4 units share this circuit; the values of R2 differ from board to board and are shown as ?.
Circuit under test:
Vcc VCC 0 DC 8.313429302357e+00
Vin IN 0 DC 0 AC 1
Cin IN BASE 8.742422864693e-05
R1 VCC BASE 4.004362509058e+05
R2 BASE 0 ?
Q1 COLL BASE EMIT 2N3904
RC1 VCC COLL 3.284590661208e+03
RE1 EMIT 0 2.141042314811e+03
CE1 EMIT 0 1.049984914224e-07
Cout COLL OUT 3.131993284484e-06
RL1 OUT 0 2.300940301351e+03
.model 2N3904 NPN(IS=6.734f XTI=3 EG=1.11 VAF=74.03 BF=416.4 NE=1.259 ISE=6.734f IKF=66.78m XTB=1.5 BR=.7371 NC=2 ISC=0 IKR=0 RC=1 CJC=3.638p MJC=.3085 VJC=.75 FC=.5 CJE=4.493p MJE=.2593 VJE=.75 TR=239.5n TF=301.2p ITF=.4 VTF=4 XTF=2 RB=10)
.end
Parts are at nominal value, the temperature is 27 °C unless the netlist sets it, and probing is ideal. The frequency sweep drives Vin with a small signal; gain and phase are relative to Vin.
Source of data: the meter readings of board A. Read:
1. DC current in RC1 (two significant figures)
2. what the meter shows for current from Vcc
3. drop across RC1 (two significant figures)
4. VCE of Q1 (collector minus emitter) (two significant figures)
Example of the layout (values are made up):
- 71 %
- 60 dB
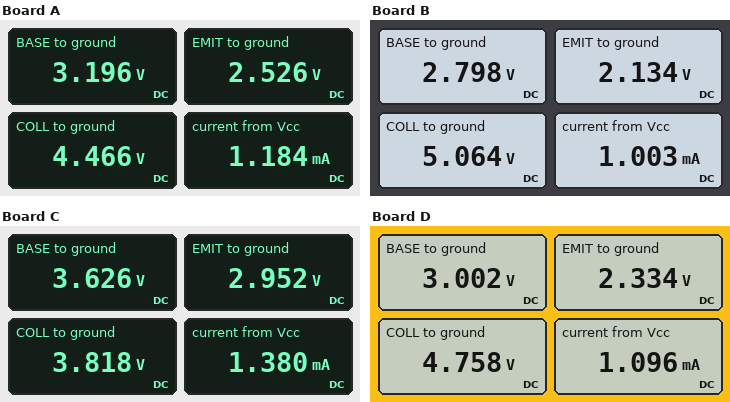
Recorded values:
- 1.2 mA
- 1.184 mA
- 3.8 V
- 1.9 V
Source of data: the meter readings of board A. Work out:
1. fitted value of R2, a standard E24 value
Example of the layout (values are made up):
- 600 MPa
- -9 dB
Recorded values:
- 750 kΩ
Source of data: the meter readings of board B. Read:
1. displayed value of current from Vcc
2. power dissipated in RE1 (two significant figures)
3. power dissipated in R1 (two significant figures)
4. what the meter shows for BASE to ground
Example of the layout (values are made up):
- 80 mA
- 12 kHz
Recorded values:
- 1.003 mA
- 2.1 mW
- 76 µW
- 2.798 V
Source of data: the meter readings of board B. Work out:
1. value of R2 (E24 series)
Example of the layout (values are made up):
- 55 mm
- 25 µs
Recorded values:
- 430 kΩ
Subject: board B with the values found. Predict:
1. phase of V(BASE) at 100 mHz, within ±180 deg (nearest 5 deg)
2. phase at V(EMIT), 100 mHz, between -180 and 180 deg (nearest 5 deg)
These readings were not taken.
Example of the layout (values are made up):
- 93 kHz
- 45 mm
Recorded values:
- 10 deg
- 10 deg
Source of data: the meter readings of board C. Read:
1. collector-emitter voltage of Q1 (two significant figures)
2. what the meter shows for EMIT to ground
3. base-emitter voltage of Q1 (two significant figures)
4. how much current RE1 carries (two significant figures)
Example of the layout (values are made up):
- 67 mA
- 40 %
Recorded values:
- 870 mV
- 2.952 V
- 670 mV
- 1.4 mA
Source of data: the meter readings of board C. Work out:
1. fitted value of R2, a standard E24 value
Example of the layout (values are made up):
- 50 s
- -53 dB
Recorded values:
- 2 MΩ
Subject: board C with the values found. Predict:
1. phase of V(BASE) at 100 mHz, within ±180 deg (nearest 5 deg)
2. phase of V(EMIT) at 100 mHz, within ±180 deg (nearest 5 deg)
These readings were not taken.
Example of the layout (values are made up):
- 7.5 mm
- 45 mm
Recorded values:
- 5 deg
- 5 deg
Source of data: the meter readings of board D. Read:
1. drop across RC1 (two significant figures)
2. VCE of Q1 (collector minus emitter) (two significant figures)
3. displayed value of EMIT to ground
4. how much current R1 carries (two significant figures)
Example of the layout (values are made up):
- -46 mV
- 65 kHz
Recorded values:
- 3.6 V
- 2.4 V
- 2.334 V
- 13 µA
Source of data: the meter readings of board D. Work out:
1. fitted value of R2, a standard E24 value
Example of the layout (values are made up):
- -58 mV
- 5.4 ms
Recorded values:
- 560 kΩ
